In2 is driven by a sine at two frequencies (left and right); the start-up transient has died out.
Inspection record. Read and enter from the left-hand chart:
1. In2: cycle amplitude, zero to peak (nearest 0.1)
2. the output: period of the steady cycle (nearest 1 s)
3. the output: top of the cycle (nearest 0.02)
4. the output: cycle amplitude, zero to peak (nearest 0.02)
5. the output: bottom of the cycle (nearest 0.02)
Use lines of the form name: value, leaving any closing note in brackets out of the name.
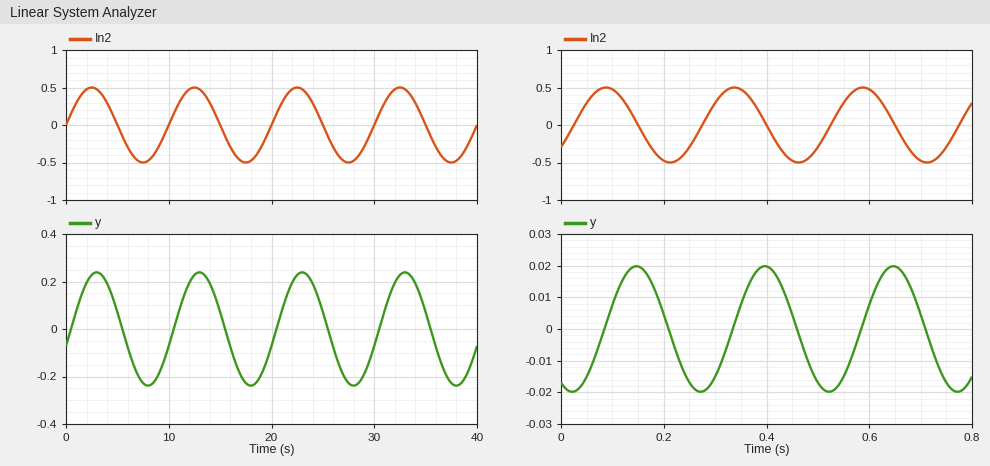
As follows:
In2: cycle amplitude, zero to peak: 0.5
the output: period of the steady cycle: 10 s
the output: top of the cycle: 0.24
the output: cycle amplitude, zero to peak: 0.24
the output: bottom of the cycle: -0.24
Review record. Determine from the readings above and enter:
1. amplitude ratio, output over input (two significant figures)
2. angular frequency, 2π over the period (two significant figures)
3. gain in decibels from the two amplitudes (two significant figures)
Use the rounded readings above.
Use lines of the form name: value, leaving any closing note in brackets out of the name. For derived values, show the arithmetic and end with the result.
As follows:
amplitude ratio, output over input: 0.24 / 0.5 = 0.48
angular frequency, 2π over the period: 2π / 10 = 0.63 rad/s
gain in decibels from the two amplitudes: 20 log10(0.24 / 0.5) = -6.4 dB
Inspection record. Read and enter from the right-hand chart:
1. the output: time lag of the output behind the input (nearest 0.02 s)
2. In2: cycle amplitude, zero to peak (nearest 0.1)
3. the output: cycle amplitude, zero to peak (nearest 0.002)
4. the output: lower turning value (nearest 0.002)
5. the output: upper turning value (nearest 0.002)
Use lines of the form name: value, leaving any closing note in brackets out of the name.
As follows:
the output: time lag of the output behind the input: 0.06 s
In2: cycle amplitude, zero to peak: 0.5
the output: cycle amplitude, zero to peak: 0.020
the output: lower turning value: -0.020
the output: upper turning value: 0.020
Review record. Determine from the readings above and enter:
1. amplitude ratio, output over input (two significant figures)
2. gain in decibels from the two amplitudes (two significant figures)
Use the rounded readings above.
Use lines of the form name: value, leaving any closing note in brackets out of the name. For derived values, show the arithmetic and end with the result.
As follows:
amplitude ratio, output over input: 0.02 / 0.5 = 0.040
gain in decibels from the two amplitudes: 20 log10(0.02 / 0.5) = -28 dB
